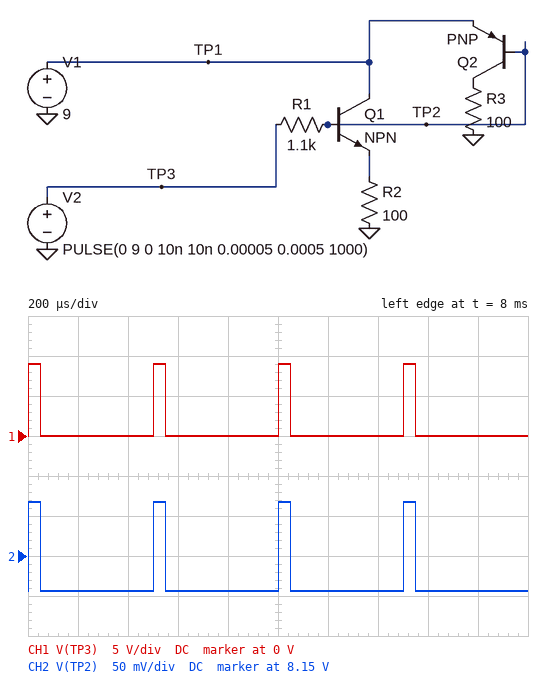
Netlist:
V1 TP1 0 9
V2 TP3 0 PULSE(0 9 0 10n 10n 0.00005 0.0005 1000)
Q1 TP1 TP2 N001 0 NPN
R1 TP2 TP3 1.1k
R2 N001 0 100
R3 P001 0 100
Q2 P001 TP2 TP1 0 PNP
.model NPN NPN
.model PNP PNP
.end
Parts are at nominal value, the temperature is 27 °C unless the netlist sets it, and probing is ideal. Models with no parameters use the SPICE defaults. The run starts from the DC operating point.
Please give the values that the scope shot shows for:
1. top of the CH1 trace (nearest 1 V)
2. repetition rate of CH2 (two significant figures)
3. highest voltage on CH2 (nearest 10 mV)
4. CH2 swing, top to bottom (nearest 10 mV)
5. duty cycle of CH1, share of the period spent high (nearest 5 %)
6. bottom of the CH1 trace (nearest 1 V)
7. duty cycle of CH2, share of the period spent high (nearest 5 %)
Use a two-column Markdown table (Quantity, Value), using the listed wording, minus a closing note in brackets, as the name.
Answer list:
| Quantity | Value |
|---|---|
| top of the CH1 trace | 9 V |
| repetition rate of CH2 | 2.0 kHz |
| highest voltage on CH2 | 8.22 V |
| CH2 swing, top to bottom | 110 mV |
| duty cycle of CH1, share of the period spent high | 10 % |
| bottom of the CH1 trace | 0 V |
| duty cycle of CH2, share of the period spent high | 10 % |
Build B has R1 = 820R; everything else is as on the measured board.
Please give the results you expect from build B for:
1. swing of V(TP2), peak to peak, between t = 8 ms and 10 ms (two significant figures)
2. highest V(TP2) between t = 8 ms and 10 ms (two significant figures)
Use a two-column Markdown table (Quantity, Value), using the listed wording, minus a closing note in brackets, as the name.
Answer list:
| Quantity | Value |
|---|---|
| swing of V(TP2), peak to peak, between t = 8 ms and 10 ms | 290 mV |
| highest V(TP2) between t = 8 ms and 10 ms | 8.4 V |
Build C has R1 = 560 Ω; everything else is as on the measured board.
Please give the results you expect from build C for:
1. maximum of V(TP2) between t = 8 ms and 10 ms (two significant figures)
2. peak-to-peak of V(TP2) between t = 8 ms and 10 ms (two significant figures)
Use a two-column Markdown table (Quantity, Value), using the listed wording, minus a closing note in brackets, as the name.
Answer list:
| Quantity | Value |
|---|---|
| maximum of V(TP2) between t = 8 ms and 10 ms | 8.6 V |
| peak-to-peak of V(TP2) between t = 8 ms and 10 ms | 470 mV |
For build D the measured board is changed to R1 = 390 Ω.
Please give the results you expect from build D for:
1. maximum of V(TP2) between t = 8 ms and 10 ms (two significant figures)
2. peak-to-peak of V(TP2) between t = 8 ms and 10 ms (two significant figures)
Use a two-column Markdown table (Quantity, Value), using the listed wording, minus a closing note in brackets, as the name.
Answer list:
| Quantity | Value |
|---|---|
| maximum of V(TP2) between t = 8 ms and 10 ms | 8.7 V |
| peak-to-peak of V(TP2) between t = 8 ms and 10 ms | 600 mV |
